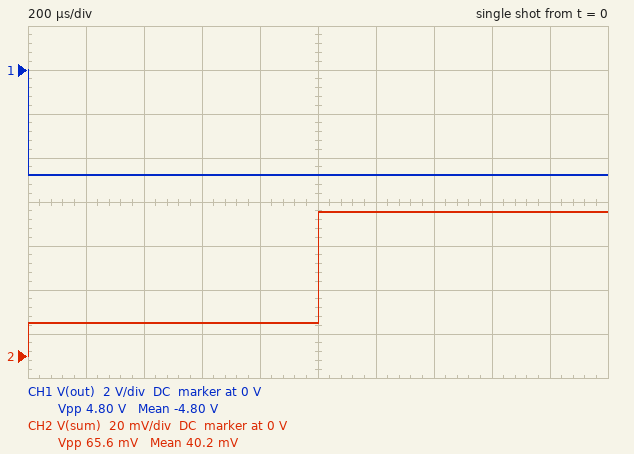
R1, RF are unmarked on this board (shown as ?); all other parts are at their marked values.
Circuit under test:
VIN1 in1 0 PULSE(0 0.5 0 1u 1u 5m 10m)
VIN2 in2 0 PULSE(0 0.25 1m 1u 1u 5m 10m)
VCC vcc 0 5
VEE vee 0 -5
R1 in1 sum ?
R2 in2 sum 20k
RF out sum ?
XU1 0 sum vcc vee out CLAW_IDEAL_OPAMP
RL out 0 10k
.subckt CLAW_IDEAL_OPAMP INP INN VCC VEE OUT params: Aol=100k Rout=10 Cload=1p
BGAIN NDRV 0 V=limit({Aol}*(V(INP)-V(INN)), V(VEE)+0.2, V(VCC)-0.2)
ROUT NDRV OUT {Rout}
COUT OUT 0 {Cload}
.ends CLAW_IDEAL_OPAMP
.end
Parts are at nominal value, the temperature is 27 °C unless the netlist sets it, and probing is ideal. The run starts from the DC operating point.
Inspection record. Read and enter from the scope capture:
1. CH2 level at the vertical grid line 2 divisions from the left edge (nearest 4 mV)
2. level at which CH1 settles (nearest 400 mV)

16 mV
-4.8 V
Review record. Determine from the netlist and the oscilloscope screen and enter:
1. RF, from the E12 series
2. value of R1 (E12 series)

56 kΩ
5.6 kΩ
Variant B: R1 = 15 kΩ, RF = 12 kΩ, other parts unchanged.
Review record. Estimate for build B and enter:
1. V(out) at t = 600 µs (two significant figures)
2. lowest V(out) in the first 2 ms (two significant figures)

-400 mV
-550 mV
